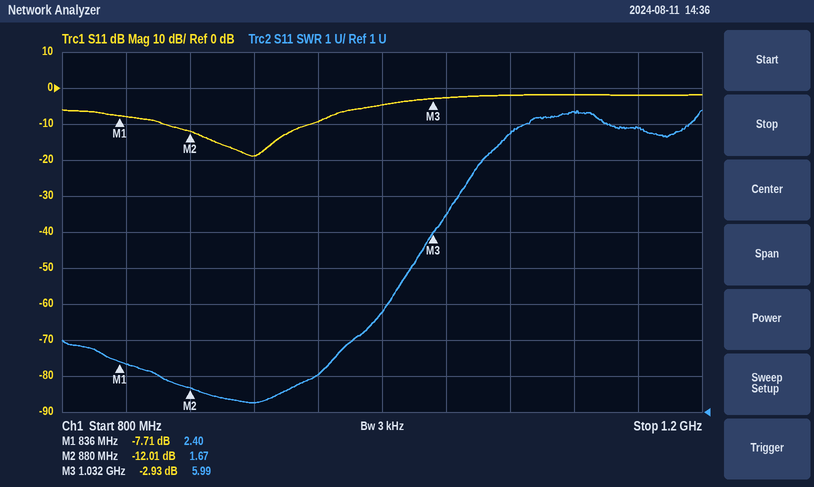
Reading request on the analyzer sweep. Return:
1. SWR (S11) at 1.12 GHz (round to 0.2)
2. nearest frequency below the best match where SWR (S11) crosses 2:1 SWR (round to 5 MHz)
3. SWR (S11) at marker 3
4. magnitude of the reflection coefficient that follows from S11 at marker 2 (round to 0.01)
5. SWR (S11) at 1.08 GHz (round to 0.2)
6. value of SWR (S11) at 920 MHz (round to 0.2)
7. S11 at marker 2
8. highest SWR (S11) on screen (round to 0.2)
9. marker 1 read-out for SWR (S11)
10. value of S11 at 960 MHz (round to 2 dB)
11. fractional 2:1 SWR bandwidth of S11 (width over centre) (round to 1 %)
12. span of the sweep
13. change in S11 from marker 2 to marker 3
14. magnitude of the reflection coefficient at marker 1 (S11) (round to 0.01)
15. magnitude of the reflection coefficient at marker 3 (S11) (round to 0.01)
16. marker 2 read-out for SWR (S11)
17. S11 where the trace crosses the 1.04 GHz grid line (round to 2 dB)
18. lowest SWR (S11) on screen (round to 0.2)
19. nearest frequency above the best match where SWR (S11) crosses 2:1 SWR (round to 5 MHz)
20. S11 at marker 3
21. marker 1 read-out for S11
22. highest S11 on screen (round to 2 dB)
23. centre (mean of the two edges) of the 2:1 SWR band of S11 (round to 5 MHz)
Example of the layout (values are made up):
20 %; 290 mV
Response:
9.4; 860 MHz; 5.99; 0.25; 8.8; 1.2; -12.01 dB; 9.4; 2.40; -10 dB; 11 %; 400 MHz; 9.08 dB; 0.41; 0.71; 1.67; -2 dB; 1.2; 960 MHz; -2.93 dB; -7.71 dB; -2 dB; 910 MHz
